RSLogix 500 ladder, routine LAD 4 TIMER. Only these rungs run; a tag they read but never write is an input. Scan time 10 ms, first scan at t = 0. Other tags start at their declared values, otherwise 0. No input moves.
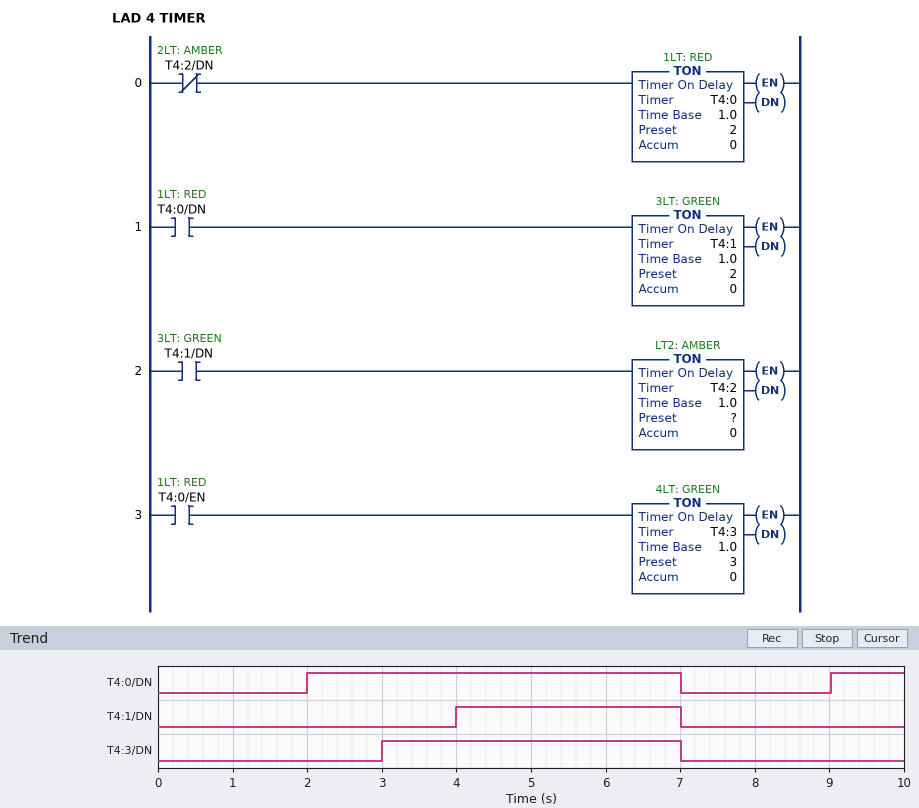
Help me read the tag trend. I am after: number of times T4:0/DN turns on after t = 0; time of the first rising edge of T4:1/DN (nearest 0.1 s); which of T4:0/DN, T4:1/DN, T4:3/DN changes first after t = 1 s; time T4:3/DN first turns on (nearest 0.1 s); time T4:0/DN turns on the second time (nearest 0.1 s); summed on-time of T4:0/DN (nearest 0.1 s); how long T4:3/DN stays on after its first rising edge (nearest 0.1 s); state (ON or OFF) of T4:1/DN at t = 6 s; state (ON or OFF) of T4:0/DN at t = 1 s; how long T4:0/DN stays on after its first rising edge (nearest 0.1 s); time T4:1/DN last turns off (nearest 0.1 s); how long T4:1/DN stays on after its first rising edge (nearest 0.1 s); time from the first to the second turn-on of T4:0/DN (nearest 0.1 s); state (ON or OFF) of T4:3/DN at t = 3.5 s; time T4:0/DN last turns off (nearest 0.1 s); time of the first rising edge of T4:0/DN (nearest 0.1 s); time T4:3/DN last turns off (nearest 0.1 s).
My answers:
2
4.0 s
T4:0/DN
3.0 s
9.0 s
6.0 s
4.0 s
ON
OFF
5.0 s
7.0 s
3.0 s
7.0 s
ON
7.0 s
2.0 s
7.0 s
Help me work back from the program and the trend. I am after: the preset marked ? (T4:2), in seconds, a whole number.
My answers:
3 s
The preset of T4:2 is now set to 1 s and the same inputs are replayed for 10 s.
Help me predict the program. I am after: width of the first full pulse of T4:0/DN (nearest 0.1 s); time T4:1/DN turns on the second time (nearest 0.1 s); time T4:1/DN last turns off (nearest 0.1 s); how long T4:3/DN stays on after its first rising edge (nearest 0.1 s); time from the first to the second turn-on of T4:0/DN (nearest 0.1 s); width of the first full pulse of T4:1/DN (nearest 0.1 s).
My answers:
3.0 s
9.0 s
5.0 s
2.0 s
5.0 s
1.0 s
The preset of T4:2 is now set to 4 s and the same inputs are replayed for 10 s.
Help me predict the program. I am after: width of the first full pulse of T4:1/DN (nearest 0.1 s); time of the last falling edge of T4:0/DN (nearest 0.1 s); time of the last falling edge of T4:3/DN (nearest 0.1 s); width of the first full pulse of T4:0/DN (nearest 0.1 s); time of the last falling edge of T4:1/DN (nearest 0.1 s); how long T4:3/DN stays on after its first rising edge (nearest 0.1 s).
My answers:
4.0 s
8.0 s
8.0 s
6.0 s
8.0 s
5.0 s
